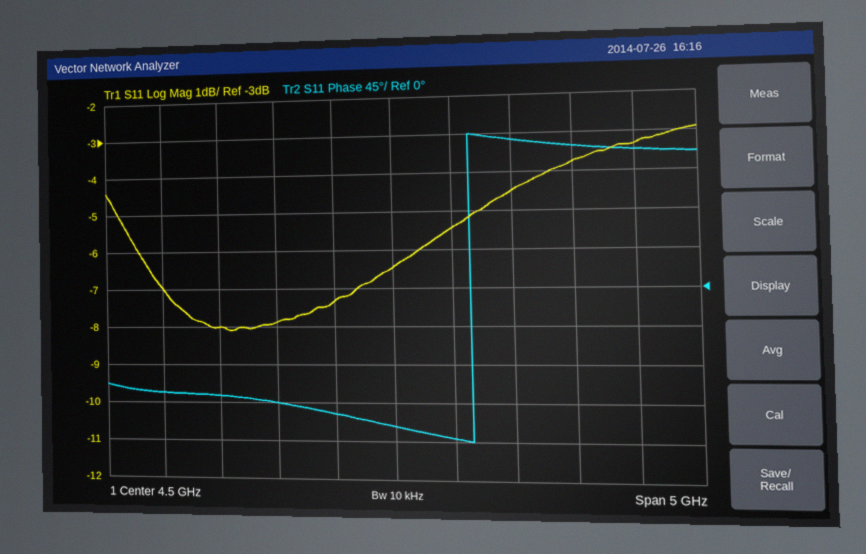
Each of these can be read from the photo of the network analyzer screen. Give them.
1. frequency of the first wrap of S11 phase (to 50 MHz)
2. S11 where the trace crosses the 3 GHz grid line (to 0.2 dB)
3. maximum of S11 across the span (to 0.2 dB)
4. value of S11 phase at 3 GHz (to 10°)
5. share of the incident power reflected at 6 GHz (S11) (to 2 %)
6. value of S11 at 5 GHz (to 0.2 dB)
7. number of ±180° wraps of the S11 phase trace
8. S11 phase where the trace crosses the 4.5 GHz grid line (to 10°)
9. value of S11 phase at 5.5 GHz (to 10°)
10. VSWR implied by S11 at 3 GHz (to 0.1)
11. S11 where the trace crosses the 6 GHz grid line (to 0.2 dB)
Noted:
5.15 GHz
-8.0 dB
-3.0 dB
-130°
42 %
-5.4 dB
1
-160°
170°
2.3
-3.8 dB
